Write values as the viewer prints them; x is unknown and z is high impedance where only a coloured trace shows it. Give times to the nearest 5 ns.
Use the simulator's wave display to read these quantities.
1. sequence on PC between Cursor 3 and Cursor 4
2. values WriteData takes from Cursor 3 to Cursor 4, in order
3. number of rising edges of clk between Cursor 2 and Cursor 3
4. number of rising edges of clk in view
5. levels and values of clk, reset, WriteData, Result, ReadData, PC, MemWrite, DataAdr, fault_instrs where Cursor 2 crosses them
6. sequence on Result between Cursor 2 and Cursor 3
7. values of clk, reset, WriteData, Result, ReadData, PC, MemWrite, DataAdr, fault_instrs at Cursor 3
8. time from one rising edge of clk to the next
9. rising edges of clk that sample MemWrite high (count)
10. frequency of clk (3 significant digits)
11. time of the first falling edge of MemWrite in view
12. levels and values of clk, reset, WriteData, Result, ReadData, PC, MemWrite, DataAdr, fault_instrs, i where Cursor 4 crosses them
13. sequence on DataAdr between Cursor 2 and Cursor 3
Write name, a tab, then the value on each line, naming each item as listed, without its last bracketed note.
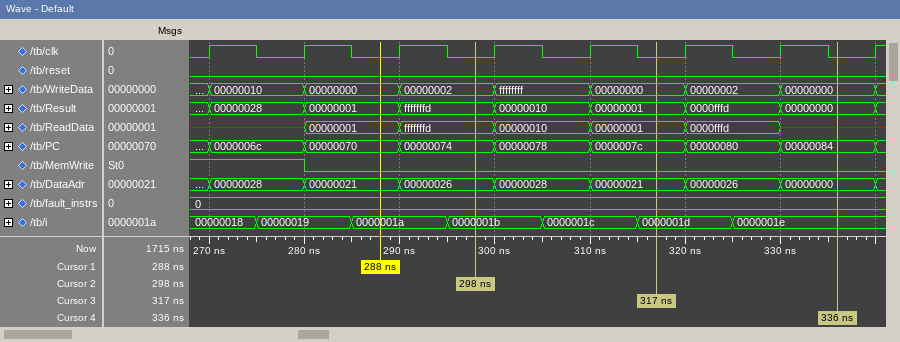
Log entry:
sequence on PC between Cursor 3 and Cursor 4	0000007c, 00000080, 00000084
values WriteData takes from Cursor 3 to Cursor 4, in order	00000000, 00000002, 00000000
number of rising edges of clk between Cursor 2 and Cursor 3	2
number of rising edges of clk in view	8
levels and values of clk, reset, WriteData, Result, ReadData, PC, MemWrite, DataAdr, fault_instrs where Cursor 2 crosses them	clk=0, reset=0, WriteData=00000002, Result=fffffffd, ReadData=fffffffd, PC=00000074, MemWrite=0, DataAdr=00000026, fault_instrs=0
sequence on Result between Cursor 2 and Cursor 3	fffffffd, 00000010, 00000001
values of clk, reset, WriteData, Result, ReadData, PC, MemWrite, DataAdr, fault_instrs at Cursor 3	clk=0, reset=0, WriteData=00000000, Result=00000001, ReadData=00000001, PC=0000007c, MemWrite=0, DataAdr=00000021, fault_instrs=0
time from one rising edge of clk to the next	10 ns
rising edges of clk that sample MemWrite high	2
frequency of clk	100 MHz
time of the first falling edge of MemWrite in view	280 ns
levels and values of clk, reset, WriteData, Result, ReadData, PC, MemWrite, DataAdr, fault_instrs, i where Cursor 4 crosses them	clk=0, reset=0, WriteData=00000000, Result=00000000, ReadData=x, PC=00000084, MemWrite=0, DataAdr=00000000, fault_instrs=0, i=0000001e
sequence on DataAdr between Cursor 2 and Cursor 3	00000026, 00000028, 00000021
